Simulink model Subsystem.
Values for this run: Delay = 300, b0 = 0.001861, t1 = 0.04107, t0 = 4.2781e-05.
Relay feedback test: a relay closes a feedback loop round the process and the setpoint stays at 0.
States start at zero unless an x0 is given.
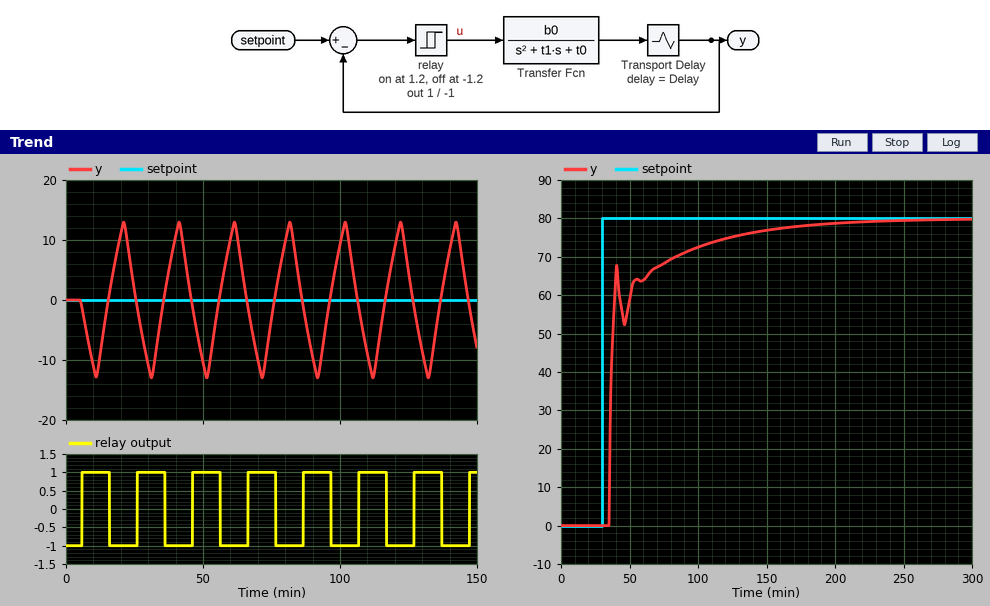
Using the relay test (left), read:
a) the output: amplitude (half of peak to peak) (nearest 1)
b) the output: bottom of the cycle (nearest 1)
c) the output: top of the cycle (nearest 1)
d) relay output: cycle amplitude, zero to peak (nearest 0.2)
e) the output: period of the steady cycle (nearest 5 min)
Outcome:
13
-13
13
1.0
20 min
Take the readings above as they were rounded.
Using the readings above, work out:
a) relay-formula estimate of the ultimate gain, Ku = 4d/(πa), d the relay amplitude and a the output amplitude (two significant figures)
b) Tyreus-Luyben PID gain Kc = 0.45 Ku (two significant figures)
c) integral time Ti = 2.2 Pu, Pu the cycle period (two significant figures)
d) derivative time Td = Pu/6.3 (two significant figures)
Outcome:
0.098
0.044
44 min
3.2 min
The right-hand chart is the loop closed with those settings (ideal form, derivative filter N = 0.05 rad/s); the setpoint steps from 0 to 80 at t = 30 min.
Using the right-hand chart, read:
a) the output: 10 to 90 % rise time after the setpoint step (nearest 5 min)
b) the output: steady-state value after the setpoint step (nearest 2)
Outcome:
60 min
80
